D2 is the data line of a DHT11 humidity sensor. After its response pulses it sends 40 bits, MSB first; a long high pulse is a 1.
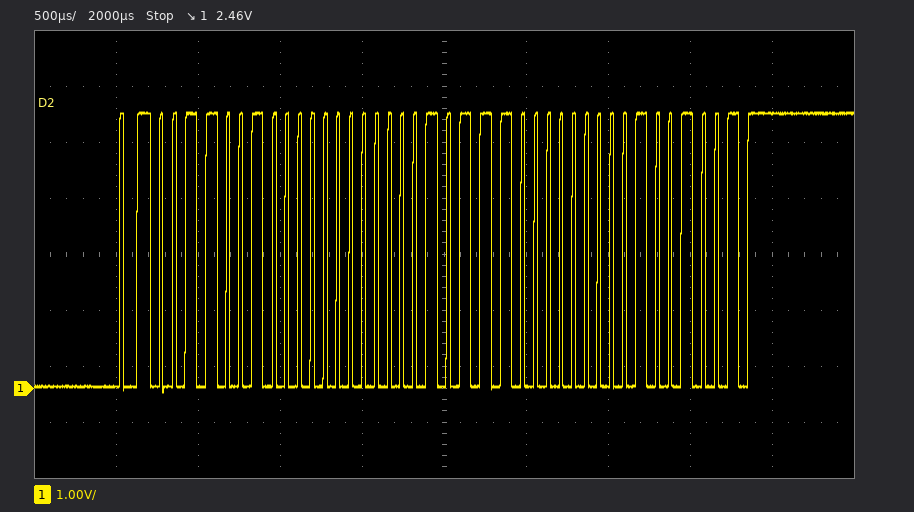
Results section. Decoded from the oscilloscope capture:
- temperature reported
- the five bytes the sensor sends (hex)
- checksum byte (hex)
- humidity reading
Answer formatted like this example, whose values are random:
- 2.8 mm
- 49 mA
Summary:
- 23.0 °C
- 32 00 17 00 49
- 0x49
- 50 %
